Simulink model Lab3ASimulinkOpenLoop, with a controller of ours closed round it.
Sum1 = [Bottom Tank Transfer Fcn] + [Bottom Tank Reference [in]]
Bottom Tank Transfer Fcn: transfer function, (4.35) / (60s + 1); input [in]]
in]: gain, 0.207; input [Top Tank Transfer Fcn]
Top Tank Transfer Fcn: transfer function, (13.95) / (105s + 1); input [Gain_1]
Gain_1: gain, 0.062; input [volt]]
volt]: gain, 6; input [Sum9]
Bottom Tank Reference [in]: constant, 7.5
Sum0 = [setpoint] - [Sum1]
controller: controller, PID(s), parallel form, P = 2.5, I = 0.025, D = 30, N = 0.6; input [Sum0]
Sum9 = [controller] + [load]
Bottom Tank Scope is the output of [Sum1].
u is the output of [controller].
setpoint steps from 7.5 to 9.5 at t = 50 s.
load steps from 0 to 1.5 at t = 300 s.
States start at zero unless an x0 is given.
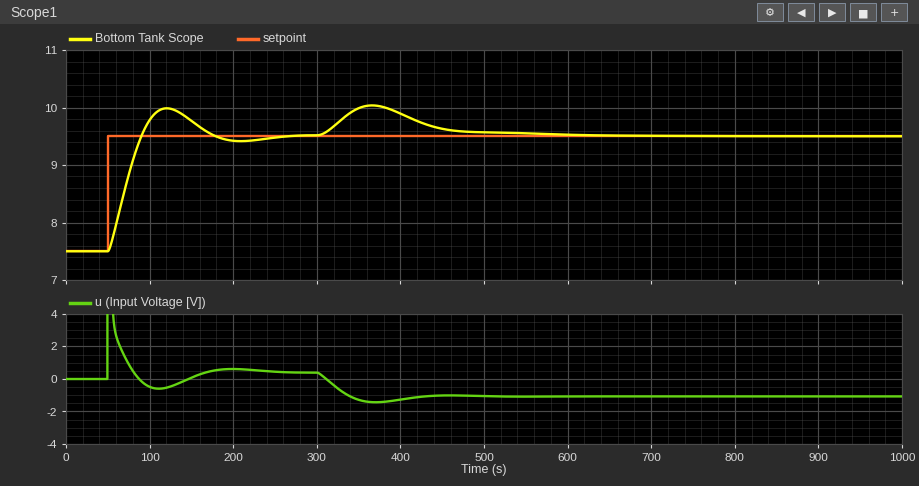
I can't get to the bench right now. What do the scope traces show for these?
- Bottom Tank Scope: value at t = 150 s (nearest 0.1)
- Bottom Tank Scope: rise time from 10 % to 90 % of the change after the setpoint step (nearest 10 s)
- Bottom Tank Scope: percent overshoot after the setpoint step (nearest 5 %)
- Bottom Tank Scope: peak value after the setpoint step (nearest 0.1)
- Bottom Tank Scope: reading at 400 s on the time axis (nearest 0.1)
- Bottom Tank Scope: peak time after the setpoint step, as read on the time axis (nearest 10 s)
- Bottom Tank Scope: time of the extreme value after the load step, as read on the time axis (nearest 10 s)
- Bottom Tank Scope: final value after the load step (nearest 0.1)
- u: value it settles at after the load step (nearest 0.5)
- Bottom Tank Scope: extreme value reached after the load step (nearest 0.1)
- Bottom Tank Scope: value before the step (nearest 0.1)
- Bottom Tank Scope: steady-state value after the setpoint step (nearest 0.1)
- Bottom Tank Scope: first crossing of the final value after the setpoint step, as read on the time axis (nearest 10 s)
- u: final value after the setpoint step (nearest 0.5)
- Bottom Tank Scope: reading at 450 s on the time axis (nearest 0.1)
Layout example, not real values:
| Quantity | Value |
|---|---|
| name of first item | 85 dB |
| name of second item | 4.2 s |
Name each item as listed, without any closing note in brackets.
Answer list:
| Quantity | Value |
|---|---|
| Bottom Tank Scope: value at t = 150 s | 9.8 |
| Bottom Tank Scope: rise time from 10 % to 90 % of the change after the setpoint step | 30 s |
| Bottom Tank Scope: percent overshoot after the setpoint step | 25 % |
| Bottom Tank Scope: peak value after the setpoint step | 10.0 |
| Bottom Tank Scope: reading at 400 s on the time axis | 9.9 |
| Bottom Tank Scope: peak time after the setpoint step, as read on the time axis | 120 s |
| Bottom Tank Scope: time of the extreme value after the load step, as read on the time axis | 370 s |
| Bottom Tank Scope: final value after the load step | 9.5 |
| u: value it settles at after the load step | -1.0 |
| Bottom Tank Scope: extreme value reached after the load step | 10.0 |
| Bottom Tank Scope: value before the step | 7.5 |
| Bottom Tank Scope: steady-state value after the setpoint step | 9.5 |
| Bottom Tank Scope: first crossing of the final value after the setpoint step, as read on the time axis | 90 s |
| u: final value after the setpoint step | 0.5 |
| Bottom Tank Scope: reading at 450 s on the time axis | 9.6 |
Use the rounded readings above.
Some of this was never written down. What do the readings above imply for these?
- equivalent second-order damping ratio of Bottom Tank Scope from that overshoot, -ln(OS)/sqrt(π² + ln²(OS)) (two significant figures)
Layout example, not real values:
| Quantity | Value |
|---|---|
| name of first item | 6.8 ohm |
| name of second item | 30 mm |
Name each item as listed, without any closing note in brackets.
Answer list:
| Quantity | Value |
|---|---|
| equivalent second-order damping ratio of Bottom Tank Scope from that overshoot, -ln(OS)/sqrt(π² + ln²(OS)) | 0.40 |
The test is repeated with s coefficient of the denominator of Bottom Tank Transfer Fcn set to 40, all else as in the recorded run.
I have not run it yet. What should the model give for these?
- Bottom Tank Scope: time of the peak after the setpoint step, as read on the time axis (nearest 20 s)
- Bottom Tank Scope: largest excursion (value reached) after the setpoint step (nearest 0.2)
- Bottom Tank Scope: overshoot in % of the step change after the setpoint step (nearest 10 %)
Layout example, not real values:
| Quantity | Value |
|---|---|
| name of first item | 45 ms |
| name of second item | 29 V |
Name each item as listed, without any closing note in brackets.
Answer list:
| Quantity | Value |
|---|---|
| Bottom Tank Scope: time of the peak after the setpoint step, as read on the time axis | 100 s |
| Bottom Tank Scope: largest excursion (value reached) after the setpoint step | 9.8 |
| Bottom Tank Scope: overshoot in % of the step change after the setpoint step | 20 % |
